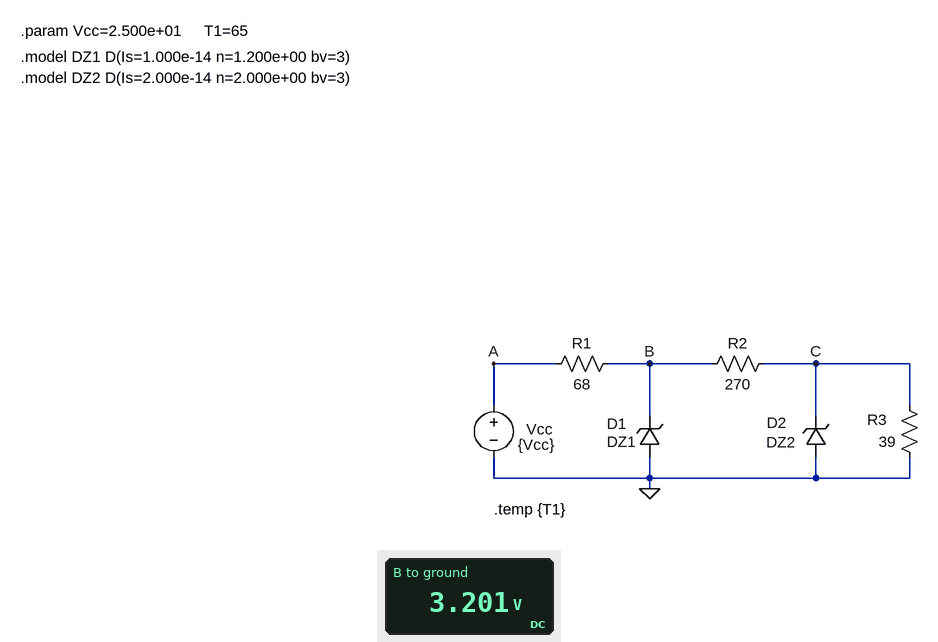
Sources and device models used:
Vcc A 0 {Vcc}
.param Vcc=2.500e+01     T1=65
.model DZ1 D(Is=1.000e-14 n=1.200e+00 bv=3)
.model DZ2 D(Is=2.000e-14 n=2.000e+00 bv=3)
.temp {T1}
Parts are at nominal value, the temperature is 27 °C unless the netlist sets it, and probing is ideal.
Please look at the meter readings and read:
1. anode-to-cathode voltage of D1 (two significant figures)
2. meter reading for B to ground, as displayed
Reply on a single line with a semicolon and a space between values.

-3.2 V; 3.201 V
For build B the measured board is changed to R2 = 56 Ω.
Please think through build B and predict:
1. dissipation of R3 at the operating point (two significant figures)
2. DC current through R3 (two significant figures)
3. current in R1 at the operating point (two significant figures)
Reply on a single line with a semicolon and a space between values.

44 mW; 34 mA; 320 mA
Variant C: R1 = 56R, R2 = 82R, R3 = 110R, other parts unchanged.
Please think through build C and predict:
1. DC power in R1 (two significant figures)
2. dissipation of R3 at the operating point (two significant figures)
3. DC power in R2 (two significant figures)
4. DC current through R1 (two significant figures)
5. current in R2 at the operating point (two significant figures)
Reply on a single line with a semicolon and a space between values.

8.5 W; 31 mW; 23 mW; 390 mA; 17 mA
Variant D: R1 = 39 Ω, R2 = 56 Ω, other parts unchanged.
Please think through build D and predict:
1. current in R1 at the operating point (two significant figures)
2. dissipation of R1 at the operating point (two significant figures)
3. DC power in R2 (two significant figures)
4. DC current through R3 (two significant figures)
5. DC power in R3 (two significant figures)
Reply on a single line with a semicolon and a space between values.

560 mA; 12 W; 64 mW; 34 mA; 45 mW
